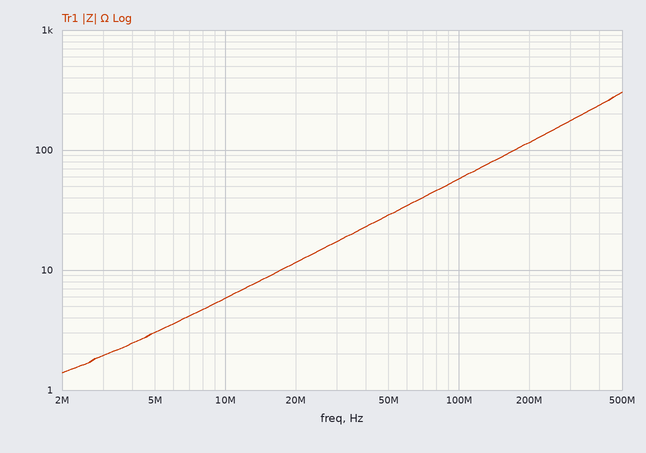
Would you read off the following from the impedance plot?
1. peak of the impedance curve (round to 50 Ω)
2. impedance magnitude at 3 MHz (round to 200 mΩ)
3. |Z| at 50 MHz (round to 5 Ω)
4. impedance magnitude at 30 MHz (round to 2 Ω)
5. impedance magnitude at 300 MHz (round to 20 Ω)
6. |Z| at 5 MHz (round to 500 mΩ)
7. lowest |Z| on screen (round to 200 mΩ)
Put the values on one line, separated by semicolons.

300 Ω; 2.0 Ω; 30 Ω; 18 Ω; 180 Ω; 3.0 Ω; 1.4 Ω
